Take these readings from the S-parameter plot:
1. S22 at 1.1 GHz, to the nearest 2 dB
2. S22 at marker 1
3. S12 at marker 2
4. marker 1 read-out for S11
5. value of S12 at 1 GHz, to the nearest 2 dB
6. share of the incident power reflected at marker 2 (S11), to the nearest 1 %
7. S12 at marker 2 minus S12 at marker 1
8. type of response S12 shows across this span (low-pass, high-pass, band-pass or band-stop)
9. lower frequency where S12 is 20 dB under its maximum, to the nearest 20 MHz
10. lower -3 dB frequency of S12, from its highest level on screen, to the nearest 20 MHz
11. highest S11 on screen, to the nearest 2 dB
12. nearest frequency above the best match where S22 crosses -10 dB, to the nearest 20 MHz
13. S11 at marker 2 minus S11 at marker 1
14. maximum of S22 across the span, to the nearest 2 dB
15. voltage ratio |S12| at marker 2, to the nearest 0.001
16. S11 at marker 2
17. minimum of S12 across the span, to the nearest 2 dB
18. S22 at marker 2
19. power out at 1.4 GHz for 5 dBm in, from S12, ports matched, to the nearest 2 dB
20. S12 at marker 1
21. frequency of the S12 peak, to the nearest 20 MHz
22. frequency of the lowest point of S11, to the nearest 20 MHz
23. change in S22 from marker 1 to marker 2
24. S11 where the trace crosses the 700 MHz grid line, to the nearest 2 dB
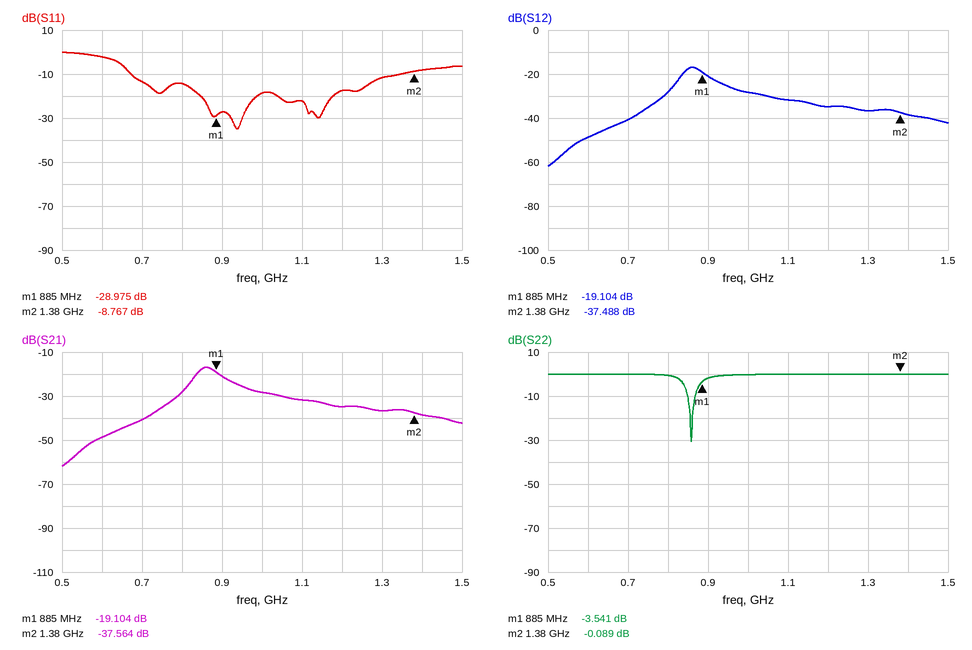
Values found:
0 dB
-3.541 dB
-37.488 dB
-28.975 dB
-28 dB
13 %
-18.384 dB
band-pass
740 MHz
840 MHz
0 dB
860 MHz
20.208 dB
0 dB
0.013
-8.767 dB
-62 dB
-0.089 dB
-34 dBm
-19.104 dB
860 MHz
940 MHz
3.452 dB
-14 dB
